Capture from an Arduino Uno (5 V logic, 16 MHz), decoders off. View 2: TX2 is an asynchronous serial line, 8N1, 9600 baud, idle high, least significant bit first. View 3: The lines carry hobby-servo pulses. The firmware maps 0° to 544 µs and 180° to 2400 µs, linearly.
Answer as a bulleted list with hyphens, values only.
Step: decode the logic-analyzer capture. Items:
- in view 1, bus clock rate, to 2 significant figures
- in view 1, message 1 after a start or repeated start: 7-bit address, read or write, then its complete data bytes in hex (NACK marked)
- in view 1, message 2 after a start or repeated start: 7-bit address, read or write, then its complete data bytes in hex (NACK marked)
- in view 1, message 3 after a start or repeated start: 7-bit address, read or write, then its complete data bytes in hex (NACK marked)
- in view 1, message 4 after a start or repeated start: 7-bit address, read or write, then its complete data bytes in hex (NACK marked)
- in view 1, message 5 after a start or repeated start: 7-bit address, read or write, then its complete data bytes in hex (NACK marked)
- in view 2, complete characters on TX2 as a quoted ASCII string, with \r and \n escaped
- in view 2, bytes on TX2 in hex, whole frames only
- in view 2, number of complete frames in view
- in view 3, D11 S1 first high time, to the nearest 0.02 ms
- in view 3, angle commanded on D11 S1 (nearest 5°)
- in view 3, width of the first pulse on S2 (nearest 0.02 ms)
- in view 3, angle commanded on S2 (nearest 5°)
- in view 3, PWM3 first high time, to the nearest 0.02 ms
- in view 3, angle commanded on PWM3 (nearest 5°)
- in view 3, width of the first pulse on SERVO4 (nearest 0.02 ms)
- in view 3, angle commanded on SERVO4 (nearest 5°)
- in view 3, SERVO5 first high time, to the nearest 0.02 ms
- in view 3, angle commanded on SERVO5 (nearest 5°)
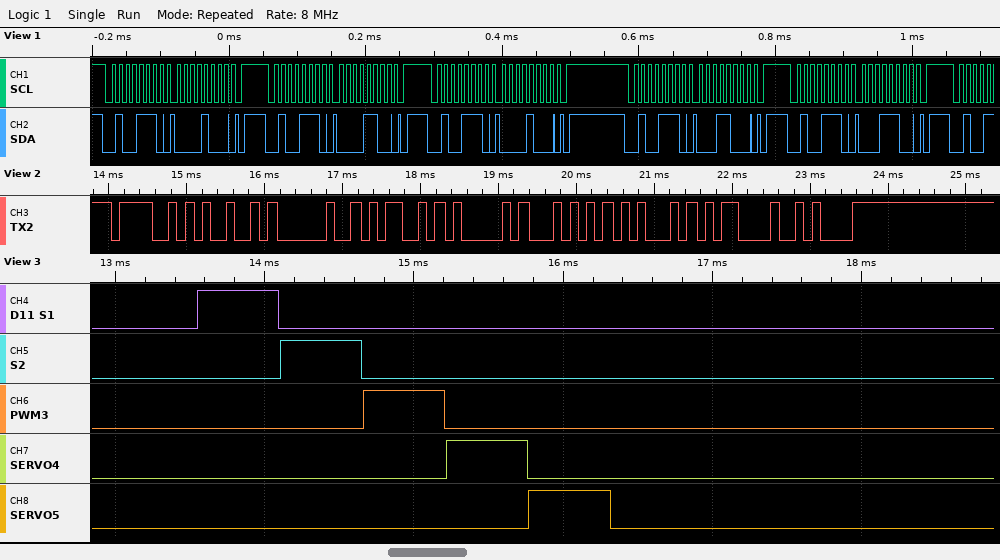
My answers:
- 100 kHz
- 0x27 write: 08
- 0x27 write: 0C
- 0x27 write: 08
- 0x27 write: 18
- 0x27 write: 1C
- "OI MATE\r\n"
- 4F 49 20 4D 41 54 45 0D 0A
- 9
- 0.54 ms
- 0°
- 0.54 ms
- 0°
- 0.54 ms
- 0°
- 0.54 ms
- 0°
- 0.54 ms
- 0°
